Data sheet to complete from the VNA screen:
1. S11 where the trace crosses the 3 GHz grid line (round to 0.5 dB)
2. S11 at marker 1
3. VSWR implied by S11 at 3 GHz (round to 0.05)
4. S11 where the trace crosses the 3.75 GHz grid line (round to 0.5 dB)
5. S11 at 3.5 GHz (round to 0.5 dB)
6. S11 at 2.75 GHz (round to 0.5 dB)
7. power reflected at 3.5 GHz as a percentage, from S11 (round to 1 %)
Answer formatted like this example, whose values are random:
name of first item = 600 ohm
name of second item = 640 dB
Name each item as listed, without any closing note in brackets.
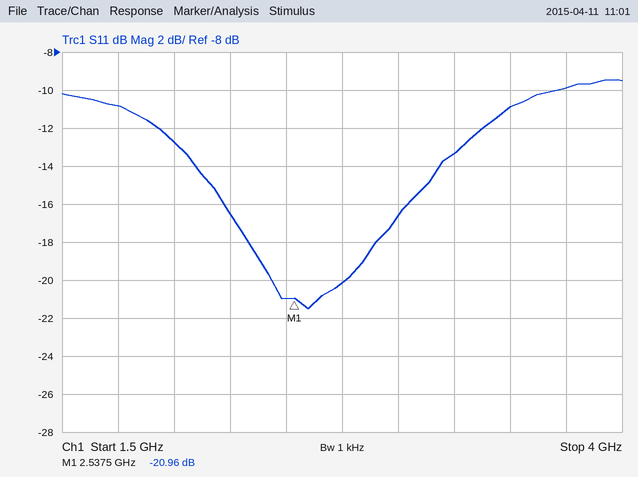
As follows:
S11 where the trace crosses the 3 GHz grid line = -16.5 dB
S11 at marker 1 = -20.96 dB
VSWR implied by S11 at 3 GHz = 1.35
S11 where the trace crosses the 3.75 GHz grid line = -10.0 dB
S11 at 3.5 GHz = -11.0 dB
S11 at 2.75 GHz = -20.0 dB
power reflected at 3.5 GHz as a percentage, from S11 = 8 %
